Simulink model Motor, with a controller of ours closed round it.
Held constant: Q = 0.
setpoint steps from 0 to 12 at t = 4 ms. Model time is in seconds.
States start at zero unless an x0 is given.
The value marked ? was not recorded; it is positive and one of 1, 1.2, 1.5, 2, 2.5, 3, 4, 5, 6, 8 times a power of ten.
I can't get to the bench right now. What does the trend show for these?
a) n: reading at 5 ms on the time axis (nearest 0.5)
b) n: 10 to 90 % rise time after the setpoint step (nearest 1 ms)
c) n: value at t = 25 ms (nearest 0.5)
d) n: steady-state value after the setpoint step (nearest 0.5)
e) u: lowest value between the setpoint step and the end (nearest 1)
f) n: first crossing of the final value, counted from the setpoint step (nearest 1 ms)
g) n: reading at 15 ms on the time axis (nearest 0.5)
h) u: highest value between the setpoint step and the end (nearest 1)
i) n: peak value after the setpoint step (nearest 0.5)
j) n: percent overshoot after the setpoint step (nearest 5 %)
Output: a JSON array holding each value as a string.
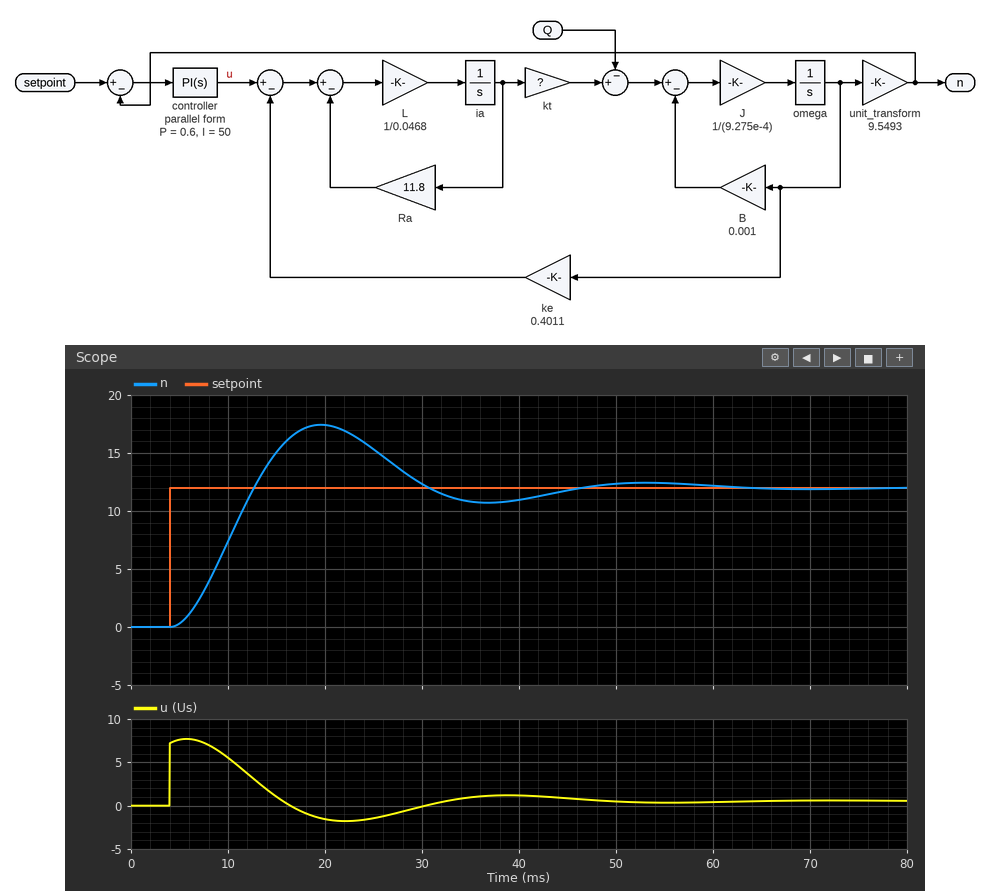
["0.5", "6 ms", "15.5", "12.0", "-2", "9 ms", "15.0", "8", "17.5", "45 %"]
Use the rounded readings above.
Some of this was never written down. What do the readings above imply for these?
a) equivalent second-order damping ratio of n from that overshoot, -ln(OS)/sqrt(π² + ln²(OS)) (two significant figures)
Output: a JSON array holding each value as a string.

["0.25"]
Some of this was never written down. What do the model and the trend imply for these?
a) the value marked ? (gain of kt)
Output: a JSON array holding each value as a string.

["0.4"]
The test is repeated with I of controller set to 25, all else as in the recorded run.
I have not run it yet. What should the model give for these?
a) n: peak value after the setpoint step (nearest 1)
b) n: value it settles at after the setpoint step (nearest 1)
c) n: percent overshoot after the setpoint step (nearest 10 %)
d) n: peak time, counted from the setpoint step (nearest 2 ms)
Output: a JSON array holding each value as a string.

["15", "12", "30 %", "16 ms"]
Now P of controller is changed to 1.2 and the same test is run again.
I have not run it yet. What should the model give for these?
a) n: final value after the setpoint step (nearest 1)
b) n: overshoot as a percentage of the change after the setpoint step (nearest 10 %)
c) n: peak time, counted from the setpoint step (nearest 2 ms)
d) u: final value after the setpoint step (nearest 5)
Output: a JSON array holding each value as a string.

["12", "40 %", "10 ms", "0"]
